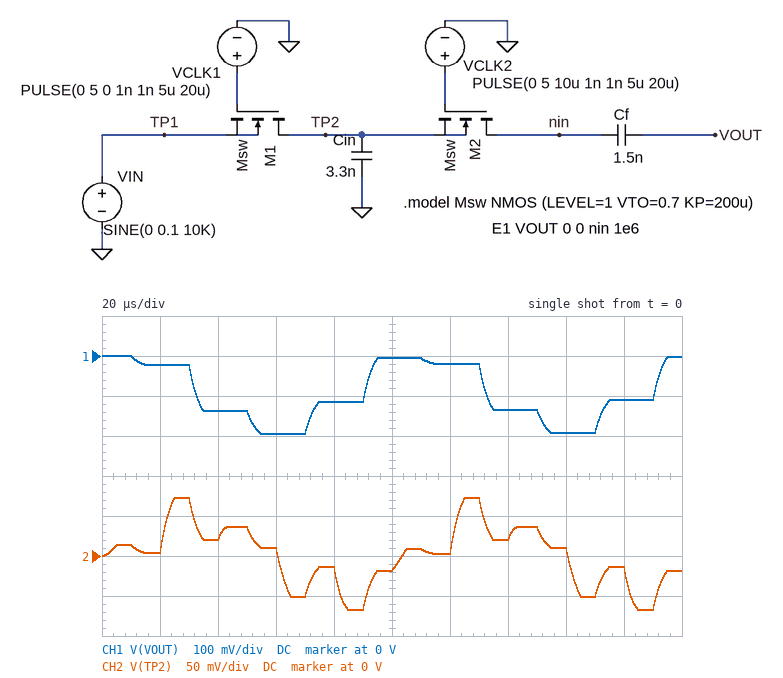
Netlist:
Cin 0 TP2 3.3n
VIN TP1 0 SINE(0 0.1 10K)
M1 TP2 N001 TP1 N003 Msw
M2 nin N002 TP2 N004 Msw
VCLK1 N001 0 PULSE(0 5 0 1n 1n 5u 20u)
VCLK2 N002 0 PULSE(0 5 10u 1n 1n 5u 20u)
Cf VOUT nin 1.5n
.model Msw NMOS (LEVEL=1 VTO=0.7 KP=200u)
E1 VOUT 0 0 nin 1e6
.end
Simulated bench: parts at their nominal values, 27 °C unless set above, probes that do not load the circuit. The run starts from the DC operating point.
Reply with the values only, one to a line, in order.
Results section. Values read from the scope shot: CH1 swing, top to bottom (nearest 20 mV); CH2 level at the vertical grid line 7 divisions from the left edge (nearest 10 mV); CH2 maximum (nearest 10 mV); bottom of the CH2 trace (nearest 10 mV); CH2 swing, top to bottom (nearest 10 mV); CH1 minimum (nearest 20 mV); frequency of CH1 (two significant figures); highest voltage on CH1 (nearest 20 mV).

200 mV
20 mV
70 mV
-70 mV
140 mV
-200 mV
10 kHz
0 V
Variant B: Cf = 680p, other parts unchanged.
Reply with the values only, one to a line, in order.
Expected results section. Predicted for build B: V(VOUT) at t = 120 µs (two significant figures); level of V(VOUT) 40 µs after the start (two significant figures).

-43 mV
-300 mV
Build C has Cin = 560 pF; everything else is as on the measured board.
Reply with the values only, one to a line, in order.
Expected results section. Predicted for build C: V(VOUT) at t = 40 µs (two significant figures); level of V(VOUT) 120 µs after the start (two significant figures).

-47 mV
-10 mV
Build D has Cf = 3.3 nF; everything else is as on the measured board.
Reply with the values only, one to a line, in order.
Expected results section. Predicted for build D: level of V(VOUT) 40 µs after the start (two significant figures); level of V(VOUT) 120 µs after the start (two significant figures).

-63 mV
-8.9 mV
